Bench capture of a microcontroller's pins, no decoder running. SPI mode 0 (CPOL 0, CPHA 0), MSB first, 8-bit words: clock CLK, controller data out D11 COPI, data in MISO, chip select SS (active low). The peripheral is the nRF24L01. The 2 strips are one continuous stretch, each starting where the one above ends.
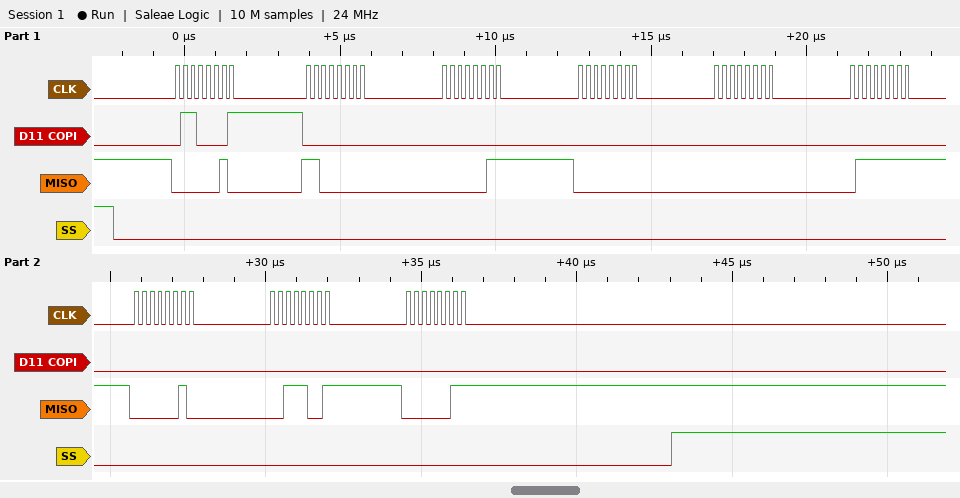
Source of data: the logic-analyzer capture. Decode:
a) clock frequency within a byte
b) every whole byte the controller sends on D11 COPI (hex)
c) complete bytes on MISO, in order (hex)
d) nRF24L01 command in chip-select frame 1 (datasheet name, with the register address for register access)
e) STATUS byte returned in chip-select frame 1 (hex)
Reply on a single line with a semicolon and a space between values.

4 MHz; 61 00 00 00 00 00 00 00 00; 02 C0 03 00 00 7F 02 39 03; R_RX_PAYLOAD; 0x02
